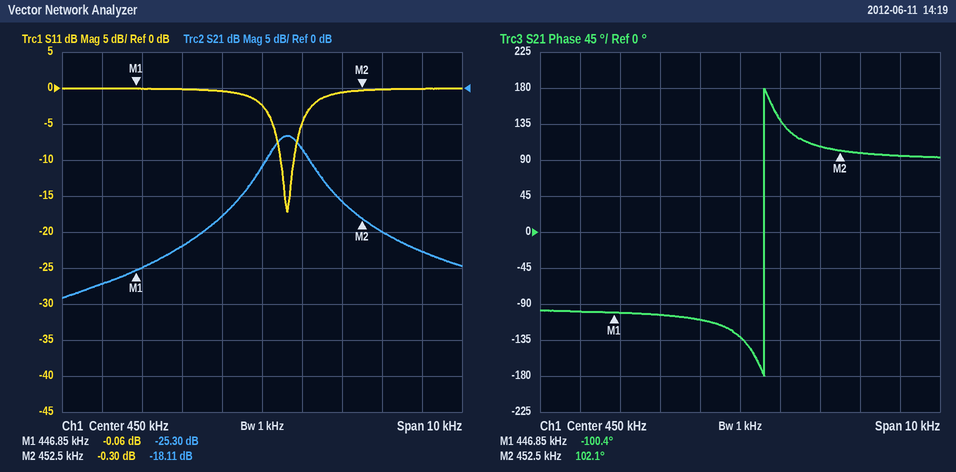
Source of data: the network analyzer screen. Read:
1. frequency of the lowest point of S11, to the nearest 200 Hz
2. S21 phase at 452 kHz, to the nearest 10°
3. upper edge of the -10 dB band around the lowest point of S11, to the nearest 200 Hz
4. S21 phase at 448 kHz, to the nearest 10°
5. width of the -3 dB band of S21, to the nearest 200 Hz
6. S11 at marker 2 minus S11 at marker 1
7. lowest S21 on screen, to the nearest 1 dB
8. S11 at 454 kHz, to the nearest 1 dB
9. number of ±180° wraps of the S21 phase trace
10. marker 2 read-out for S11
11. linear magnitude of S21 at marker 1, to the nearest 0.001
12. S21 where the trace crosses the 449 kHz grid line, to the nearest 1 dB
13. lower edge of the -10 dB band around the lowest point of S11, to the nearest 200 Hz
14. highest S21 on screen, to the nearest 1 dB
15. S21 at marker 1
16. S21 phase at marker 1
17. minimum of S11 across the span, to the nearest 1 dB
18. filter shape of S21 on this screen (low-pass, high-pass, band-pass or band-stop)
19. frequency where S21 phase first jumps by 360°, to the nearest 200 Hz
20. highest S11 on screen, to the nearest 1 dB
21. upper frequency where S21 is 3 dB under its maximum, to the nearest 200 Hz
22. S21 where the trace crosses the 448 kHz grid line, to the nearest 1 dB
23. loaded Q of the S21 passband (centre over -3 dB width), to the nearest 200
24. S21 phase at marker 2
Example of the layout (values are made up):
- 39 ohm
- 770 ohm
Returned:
- 450.6 kHz
- 110°
- 450.8 kHz
- -100°
- 1.0 kHz
- -0.24 dB
- -29 dB
- 0 dB
- 1
- -0.30 dB
- 0.054
- -18 dB
- 450.4 kHz
- -7 dB
- -25.30 dB
- -100.4°
- -17 dB
- band-pass
- 450.6 kHz
- 0 dB
- 451.2 kHz
- -22 dB
- 400
- 102.1°
